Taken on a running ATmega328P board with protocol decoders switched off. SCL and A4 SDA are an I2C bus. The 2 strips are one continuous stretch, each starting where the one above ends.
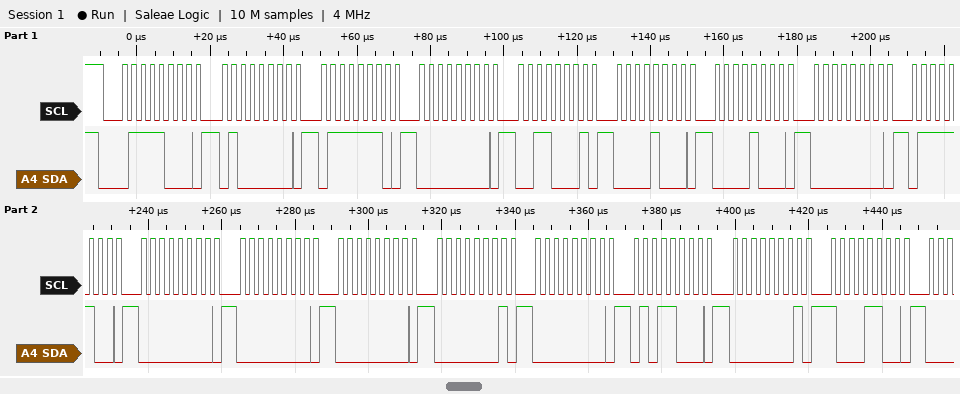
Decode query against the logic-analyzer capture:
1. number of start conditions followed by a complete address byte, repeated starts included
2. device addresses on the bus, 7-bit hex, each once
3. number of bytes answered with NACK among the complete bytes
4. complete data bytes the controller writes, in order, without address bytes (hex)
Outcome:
1
0x3C
0
40 7E 00 31 08 08 00 7C 00 00 00 01 00 58 01 8C
